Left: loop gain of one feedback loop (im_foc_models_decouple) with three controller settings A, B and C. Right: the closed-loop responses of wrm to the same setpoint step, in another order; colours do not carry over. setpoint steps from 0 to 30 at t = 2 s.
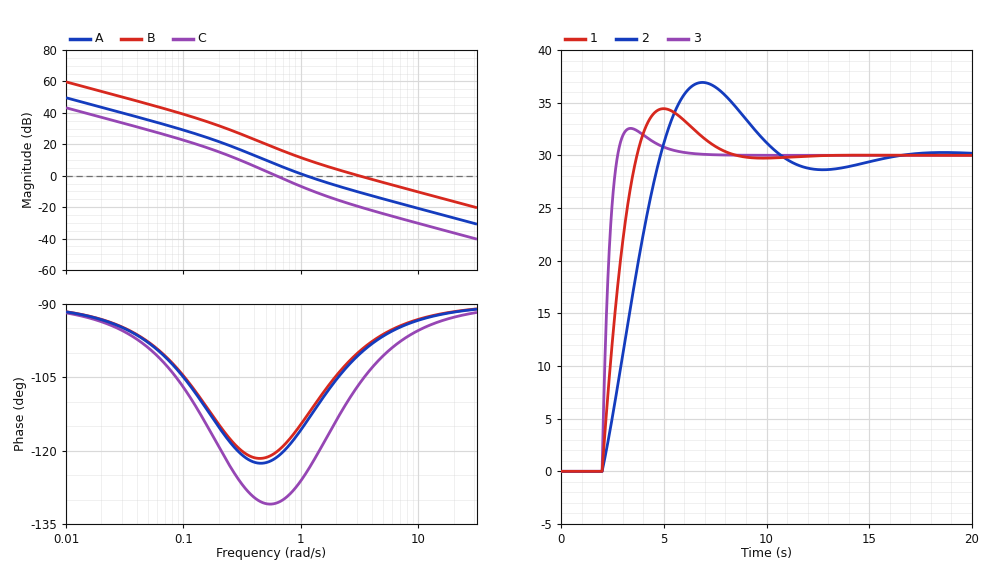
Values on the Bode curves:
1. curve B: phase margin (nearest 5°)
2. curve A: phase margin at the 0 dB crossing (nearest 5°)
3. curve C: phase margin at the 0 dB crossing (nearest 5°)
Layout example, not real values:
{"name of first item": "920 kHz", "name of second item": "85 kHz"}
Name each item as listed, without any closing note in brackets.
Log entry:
{"curve B: phase margin": "80°", "curve A: phase margin at the 0 dB crossing": "65°", "curve C: phase margin at the 0 dB crossing": "50°"}
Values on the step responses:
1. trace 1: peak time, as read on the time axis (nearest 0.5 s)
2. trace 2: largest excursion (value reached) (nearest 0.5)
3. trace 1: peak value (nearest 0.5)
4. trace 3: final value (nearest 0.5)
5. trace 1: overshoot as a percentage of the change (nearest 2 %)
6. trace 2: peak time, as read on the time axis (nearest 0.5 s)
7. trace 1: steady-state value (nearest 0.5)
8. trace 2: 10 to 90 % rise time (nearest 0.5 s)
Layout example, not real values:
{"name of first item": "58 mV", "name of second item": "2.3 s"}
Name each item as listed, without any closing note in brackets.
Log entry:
{"trace 1: peak time, as read on the time axis": "5.0 s", "trace 2: largest excursion (value reached)": "37.0", "trace 1: peak value": "34.5", "trace 3: final value": "30.0", "trace 1: overshoot as a percentage of the change": "14 %", "trace 2: peak time, as read on the time axis": "7.0 s", "trace 1: steady-state value": "30.0", "trace 2: 10 to 90 % rise time": "2.0 s"}
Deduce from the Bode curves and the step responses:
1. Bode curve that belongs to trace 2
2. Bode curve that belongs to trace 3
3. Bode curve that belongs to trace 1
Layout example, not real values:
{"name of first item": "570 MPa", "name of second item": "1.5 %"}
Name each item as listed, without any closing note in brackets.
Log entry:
{"Bode curve that belongs to trace 2": "C", "Bode curve that belongs to trace 3": "B", "Bode curve that belongs to trace 1": "A"}
